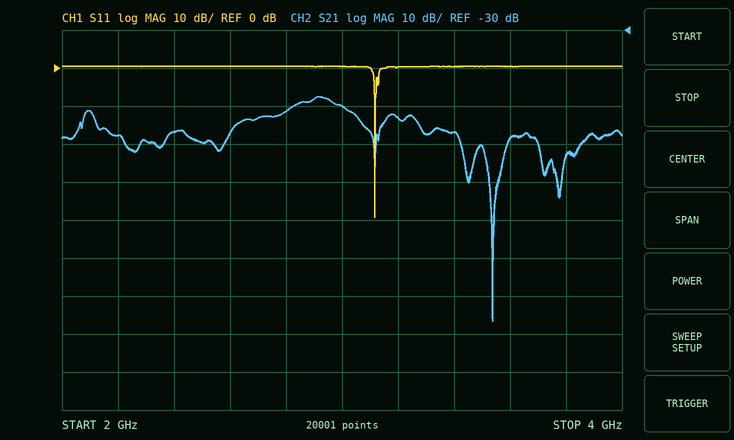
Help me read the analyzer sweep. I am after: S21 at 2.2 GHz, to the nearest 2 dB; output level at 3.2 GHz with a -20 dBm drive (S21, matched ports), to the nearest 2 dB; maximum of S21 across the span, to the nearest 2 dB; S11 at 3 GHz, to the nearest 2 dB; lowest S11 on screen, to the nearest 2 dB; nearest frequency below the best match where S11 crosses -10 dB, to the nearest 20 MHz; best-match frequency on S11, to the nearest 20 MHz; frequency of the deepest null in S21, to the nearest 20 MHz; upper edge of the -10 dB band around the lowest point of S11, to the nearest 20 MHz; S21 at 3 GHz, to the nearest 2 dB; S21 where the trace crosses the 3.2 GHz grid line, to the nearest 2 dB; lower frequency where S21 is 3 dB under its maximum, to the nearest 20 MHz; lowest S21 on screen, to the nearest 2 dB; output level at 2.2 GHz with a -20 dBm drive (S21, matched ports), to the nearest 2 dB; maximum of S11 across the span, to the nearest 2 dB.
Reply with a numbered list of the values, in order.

1. -58 dB
2. -74 dBm
3. -48 dB
4. 0 dB
5. -40 dB
6. 3.12 GHz
7. 3.12 GHz
8. 3.54 GHz
9. 3.12 GHz
10. -50 dB
11. -54 dB
12. 2.82 GHz
13. -106 dB
14. -78 dBm
15. 0 dB
